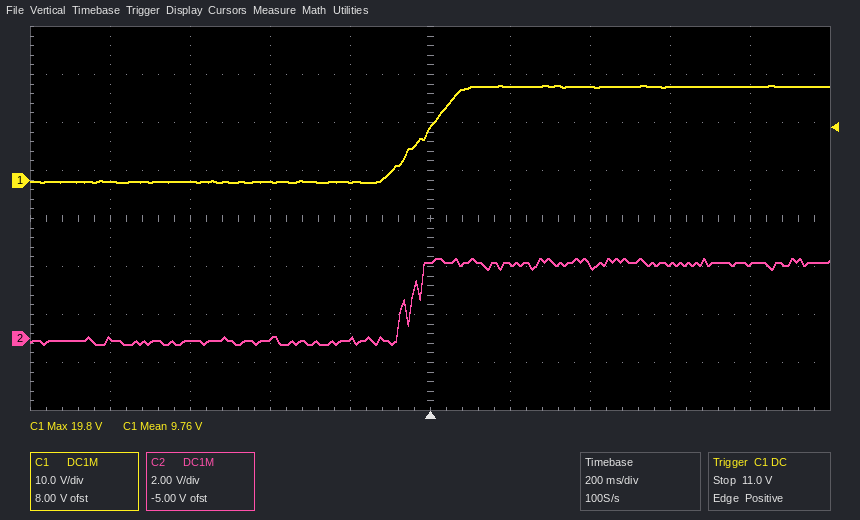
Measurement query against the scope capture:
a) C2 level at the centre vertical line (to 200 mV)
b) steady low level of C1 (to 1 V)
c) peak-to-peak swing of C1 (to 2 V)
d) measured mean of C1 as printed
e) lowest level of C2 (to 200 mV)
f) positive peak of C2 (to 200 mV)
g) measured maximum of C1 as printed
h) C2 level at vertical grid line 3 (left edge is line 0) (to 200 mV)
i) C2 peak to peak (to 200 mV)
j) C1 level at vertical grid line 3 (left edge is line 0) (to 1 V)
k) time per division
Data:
3.2 V
0 V
20 V
9.76 V
-200 mV
3.4 V
19.8 V
0.0 V
3.6 V
0 V
200 ms
